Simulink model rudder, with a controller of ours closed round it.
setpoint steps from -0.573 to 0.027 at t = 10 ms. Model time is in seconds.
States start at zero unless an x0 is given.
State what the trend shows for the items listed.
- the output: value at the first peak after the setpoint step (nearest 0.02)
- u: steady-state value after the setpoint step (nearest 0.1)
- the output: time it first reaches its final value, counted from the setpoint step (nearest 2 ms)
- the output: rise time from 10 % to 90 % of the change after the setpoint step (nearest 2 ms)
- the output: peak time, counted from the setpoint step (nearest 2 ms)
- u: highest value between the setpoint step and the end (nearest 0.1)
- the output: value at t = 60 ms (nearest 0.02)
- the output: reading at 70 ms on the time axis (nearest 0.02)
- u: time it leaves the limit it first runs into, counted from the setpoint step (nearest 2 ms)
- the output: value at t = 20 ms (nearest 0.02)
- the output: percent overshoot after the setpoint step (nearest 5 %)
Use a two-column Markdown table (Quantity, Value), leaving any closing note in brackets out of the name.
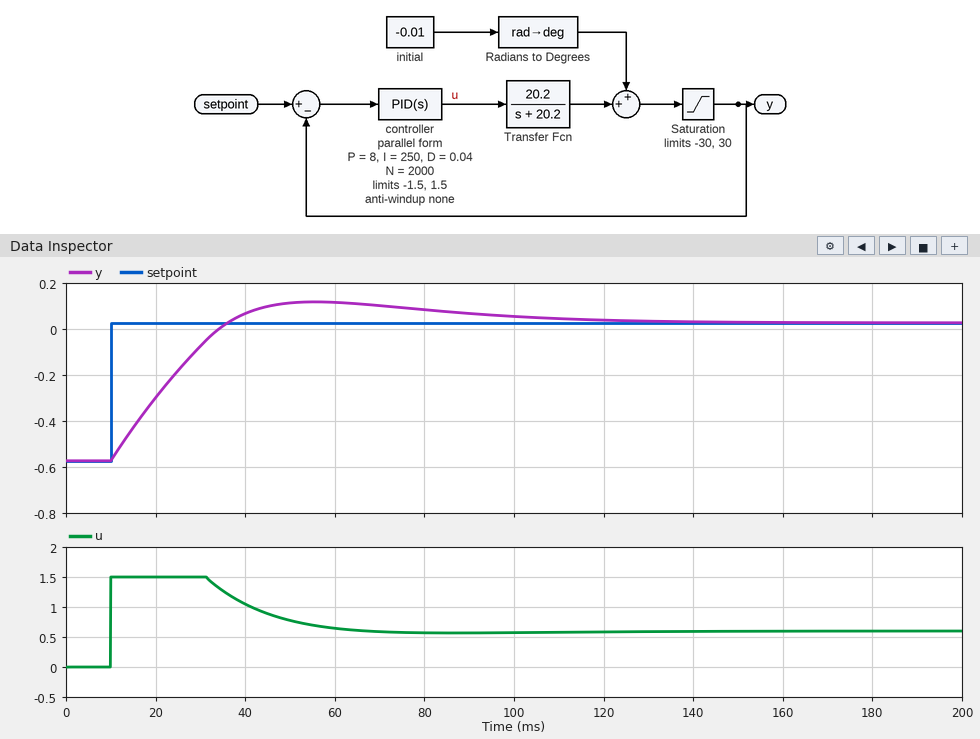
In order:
| Quantity | Value |
|---|---|
| the output: value at the first peak after the setpoint step | 0.12 |
| u: steady-state value after the setpoint step | 0.6 |
| the output: time it first reaches its final value, counted from the setpoint step | 26 ms |
| the output: rise time from 10 % to 90 % of the change after the setpoint step | 20 ms |
| the output: peak time, counted from the setpoint step | 46 ms |
| u: highest value between the setpoint step and the end | 1.5 |
| the output: value at t = 60 ms | 0.12 |
| the output: reading at 70 ms on the time axis | 0.10 |
| u: time it leaves the limit it first runs into, counted from the setpoint step | 22 ms |
| the output: value at t = 20 ms | -0.30 |
| the output: percent overshoot after the setpoint step | 15 % |
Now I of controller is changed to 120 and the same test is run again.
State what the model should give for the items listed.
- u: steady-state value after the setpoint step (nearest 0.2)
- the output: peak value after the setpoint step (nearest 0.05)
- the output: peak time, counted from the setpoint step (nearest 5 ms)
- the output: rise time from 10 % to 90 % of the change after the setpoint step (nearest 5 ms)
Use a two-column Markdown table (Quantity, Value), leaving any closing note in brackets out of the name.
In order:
| Quantity | Value |
|---|---|
| u: steady-state value after the setpoint step | 0.6 |
| the output: peak value after the setpoint step | 0.05 |
| the output: peak time, counted from the setpoint step | 60 ms |
| the output: rise time from 10 % to 90 % of the change after the setpoint step | 25 ms |
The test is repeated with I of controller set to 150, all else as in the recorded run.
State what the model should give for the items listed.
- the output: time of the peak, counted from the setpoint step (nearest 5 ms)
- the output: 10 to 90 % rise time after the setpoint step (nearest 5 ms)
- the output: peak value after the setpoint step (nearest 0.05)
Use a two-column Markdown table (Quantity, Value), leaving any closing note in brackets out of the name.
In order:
| Quantity | Value |
|---|---|
| the output: time of the peak, counted from the setpoint step | 55 ms |
| the output: 10 to 90 % rise time after the setpoint step | 20 ms |
| the output: peak value after the setpoint step | 0.05 |
